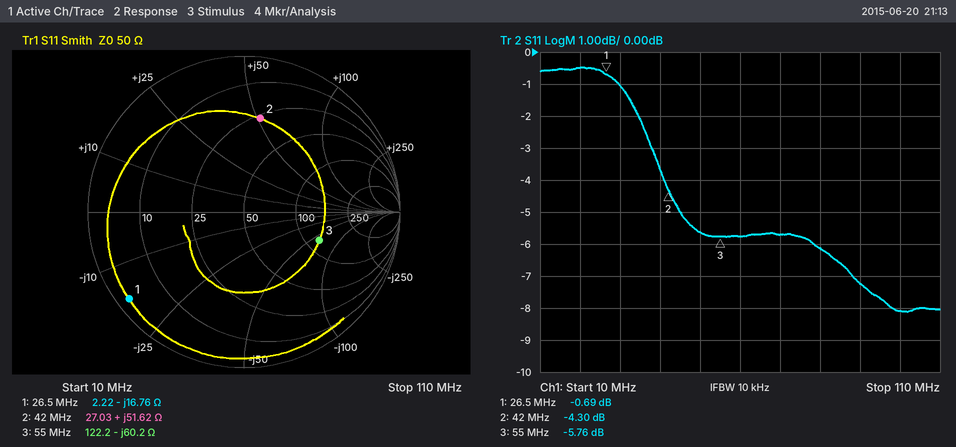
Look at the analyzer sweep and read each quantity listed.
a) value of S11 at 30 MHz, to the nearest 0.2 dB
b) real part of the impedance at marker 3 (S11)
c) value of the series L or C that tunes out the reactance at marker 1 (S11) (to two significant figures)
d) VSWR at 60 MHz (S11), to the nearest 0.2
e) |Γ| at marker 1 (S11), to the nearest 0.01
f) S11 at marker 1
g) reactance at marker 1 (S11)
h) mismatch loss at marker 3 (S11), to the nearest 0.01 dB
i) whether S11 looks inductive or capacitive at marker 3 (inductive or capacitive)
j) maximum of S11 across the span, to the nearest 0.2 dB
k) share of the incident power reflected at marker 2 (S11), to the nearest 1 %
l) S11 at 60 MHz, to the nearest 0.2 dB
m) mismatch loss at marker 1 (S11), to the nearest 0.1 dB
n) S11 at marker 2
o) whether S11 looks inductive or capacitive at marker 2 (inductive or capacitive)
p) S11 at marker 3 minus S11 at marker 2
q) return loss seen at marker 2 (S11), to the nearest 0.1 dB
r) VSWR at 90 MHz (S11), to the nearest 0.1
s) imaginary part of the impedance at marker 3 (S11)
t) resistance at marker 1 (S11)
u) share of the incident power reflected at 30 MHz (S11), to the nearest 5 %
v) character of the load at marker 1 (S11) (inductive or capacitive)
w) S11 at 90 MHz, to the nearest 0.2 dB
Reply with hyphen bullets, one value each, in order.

- -1.0 dB
- 122.2 Ω
- 100 nH
- 3.2
- 0.92
- -0.69 dB
- -16.76 Ω
- 1.34 dB
- capacitive
- -0.4 dB
- 37 %
- -5.8 dB
- 8.3 dB
- -4.30 dB
- inductive
- -1.46 dB
- 4.3 dB
- 2.5
- -60.2 Ω
- 2.22 Ω
- 80 %
- capacitive
- -7.2 dB
